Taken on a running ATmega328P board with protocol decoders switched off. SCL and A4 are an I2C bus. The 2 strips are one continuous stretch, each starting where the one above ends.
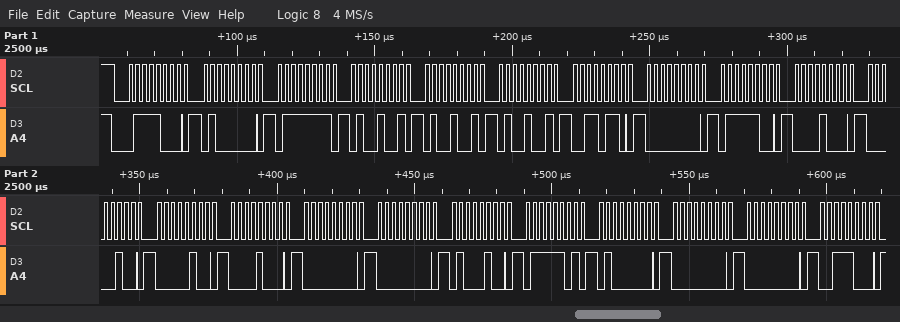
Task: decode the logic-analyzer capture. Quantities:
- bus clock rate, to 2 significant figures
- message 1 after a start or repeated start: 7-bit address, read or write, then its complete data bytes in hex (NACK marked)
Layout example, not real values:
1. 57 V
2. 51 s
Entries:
1. 400 kHz
2. 0x3C write: 40 7F 49 49 49 36 00 7C 08 04 04 08 00 00 44 7D 40 00 00 38
